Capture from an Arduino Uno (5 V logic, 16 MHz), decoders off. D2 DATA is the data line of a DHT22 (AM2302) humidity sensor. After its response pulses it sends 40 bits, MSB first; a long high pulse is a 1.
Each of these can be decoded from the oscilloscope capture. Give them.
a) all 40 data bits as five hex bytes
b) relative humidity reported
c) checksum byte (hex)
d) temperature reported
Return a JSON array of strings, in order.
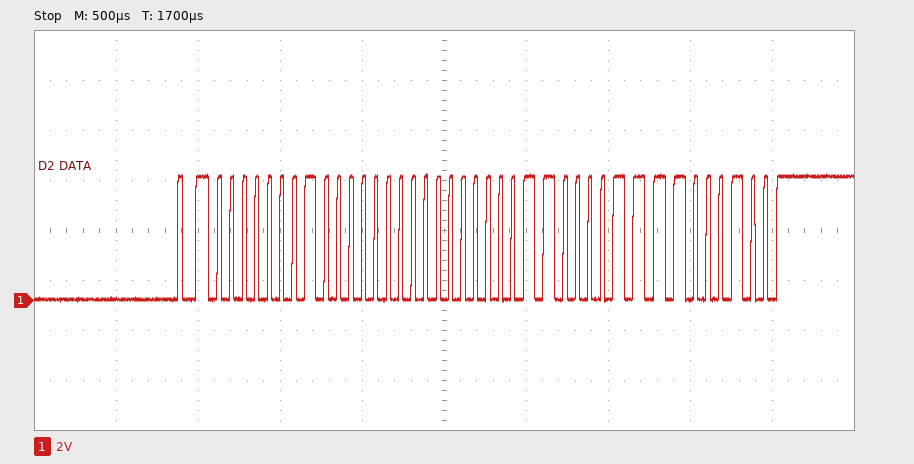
["01 00 00 C3 C4", "25.6 %", "0xC4", "19.5 °C"]
